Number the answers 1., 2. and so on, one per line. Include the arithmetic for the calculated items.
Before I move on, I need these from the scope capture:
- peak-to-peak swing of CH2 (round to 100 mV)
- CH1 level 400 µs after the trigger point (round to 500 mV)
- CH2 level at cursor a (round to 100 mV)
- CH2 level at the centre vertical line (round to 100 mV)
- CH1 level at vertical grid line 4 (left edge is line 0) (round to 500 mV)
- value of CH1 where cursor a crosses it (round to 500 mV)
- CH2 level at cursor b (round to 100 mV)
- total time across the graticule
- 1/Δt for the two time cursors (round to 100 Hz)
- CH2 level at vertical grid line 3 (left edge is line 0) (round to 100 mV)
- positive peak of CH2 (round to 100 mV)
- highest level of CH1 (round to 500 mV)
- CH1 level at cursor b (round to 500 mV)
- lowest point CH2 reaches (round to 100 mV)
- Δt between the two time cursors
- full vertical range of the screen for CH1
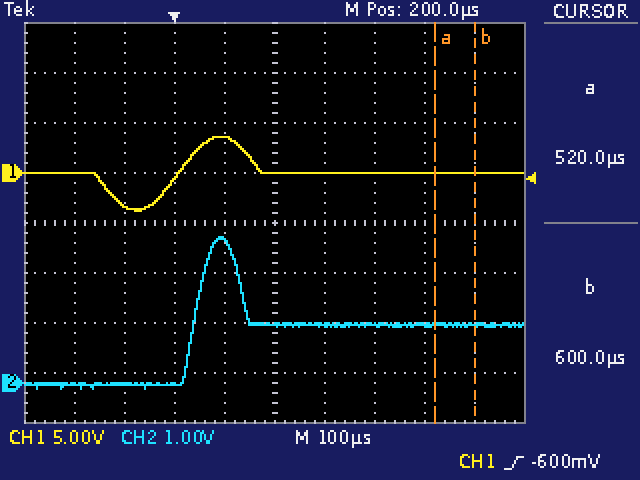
1. 2.9 V − (-100 mV) = 3.0 V
2. 0.0 V
3. 1.2 V
4. 1.2 V
5. 3.5 V
6. 0.0 V
7. 1.2 V
8. 1 ms
9. 1 / 80 µs ≈ 12.5 kHz
10. 0.0 V
11. 2.9 V
12. 3.5 V
13. 0.0 V
14. -100 mV
15. 600 µs − (520 µs) = 80 µs
16. 40 V
